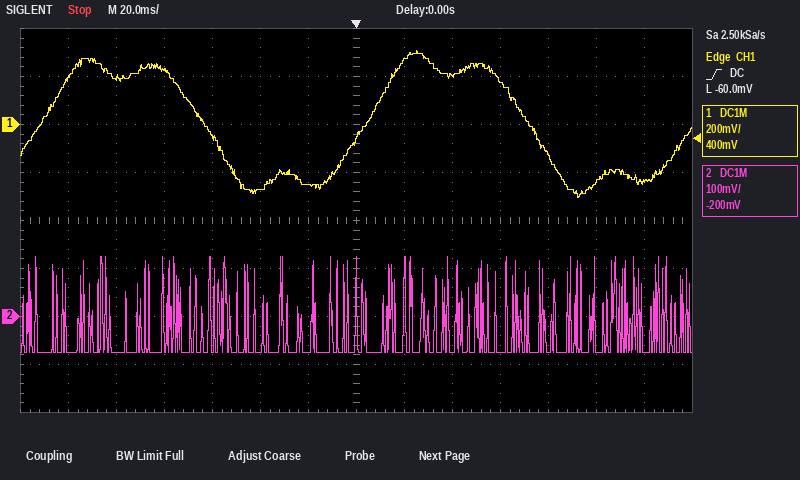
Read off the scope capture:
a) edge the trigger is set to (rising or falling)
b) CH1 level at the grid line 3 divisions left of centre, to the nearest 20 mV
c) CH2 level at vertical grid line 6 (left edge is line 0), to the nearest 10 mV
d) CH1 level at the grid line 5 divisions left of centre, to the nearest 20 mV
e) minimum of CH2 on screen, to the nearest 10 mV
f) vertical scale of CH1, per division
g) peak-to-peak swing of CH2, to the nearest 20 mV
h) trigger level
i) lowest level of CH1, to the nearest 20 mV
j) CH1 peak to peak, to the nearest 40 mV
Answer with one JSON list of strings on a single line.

["rising", "-40 mV", "-80 mV", "200 mV", "-80 mV", "200 mV", "200 mV", "-60.0 mV", "-300 mV", "600 mV"]
